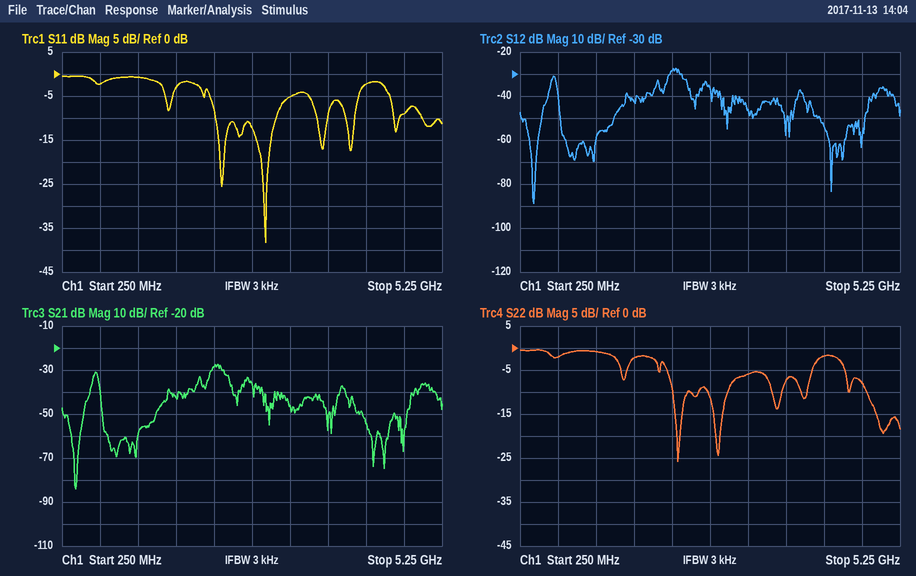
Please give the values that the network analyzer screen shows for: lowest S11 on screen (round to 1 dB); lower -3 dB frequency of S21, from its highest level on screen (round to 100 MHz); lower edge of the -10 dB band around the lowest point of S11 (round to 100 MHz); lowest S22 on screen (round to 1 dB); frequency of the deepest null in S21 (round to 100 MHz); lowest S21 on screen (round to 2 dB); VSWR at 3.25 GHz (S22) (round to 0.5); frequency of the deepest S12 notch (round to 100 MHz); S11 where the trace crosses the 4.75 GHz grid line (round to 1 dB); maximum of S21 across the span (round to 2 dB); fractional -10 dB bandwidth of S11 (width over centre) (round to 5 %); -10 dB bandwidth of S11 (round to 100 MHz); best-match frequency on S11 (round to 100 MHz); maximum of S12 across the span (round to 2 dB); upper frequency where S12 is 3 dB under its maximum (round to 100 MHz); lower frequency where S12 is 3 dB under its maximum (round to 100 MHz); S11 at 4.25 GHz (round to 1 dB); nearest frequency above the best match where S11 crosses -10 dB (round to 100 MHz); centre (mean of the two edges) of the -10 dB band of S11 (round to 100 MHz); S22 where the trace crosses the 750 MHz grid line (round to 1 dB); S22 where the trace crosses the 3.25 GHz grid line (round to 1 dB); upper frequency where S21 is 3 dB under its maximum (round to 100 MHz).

-38 dB
2.2 GHz
2.3 GHz
-26 dB
400 MHz
-84 dB
3.0
400 MHz
-9 dB
-28 dB
30 %
800 MHz
2.9 GHz
-28 dB
2.4 GHz
2.2 GHz
-2 dB
3.1 GHz
2.7 GHz
-2 dB
-6 dB
2.4 GHz
